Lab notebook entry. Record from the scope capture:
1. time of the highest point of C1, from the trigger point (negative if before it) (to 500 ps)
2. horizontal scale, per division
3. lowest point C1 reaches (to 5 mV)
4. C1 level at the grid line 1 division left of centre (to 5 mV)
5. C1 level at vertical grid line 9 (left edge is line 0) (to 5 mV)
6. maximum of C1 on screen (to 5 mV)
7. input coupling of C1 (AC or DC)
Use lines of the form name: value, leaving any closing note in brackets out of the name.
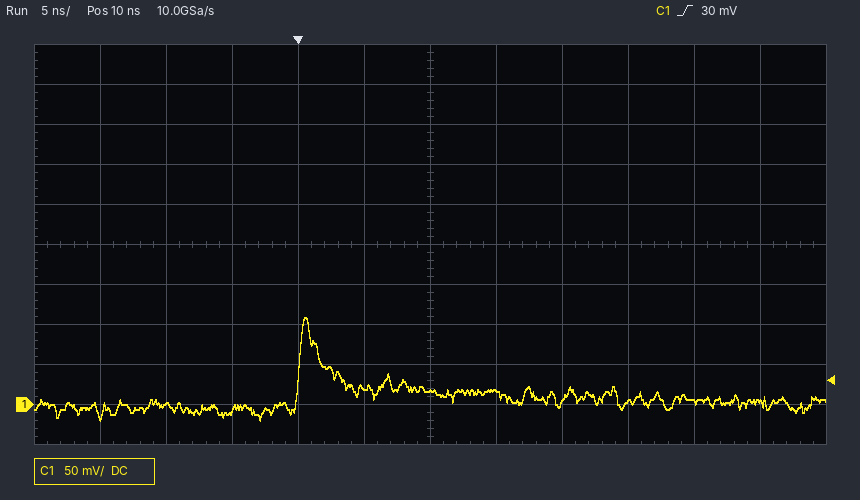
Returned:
time of the highest point of C1, from the trigger point (negative if before it): +500 ps
horizontal scale, per division: 5 ns
lowest point C1 reaches: -20 mV
C1 level at the grid line 1 division left of centre: 20 mV
C1 level at vertical grid line 9 (left edge is line 0): 5 mV
maximum of C1 on screen: 110 mV
input coupling of C1: DC
